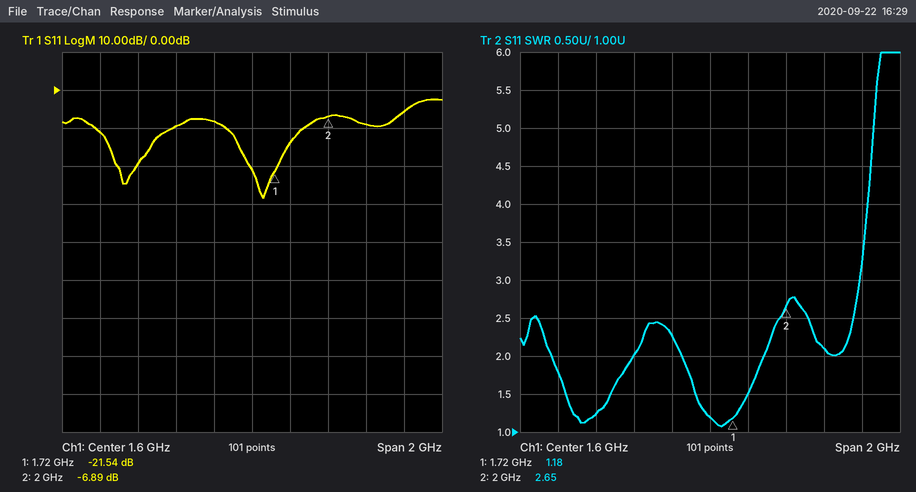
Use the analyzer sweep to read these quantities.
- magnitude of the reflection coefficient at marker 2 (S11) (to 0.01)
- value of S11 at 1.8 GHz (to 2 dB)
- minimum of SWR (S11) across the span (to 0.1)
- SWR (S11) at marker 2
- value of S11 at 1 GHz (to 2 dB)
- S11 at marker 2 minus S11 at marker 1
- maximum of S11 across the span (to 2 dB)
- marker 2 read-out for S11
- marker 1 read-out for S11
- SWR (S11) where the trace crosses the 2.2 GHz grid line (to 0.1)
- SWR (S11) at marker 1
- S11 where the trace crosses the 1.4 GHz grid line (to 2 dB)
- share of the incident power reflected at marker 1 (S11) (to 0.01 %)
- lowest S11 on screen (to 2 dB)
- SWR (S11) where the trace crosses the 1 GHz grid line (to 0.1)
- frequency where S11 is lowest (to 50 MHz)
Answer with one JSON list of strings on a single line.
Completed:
["0.45", "-14 dB", "1.1", "2.65", "-20 dB", "14.65 dB", "-2 dB", "-6.89 dB", "-21.54 dB", "2.1", "1.18", "-8 dB", "0.70 %", "-28 dB", "1.2", "1.65 GHz"]
